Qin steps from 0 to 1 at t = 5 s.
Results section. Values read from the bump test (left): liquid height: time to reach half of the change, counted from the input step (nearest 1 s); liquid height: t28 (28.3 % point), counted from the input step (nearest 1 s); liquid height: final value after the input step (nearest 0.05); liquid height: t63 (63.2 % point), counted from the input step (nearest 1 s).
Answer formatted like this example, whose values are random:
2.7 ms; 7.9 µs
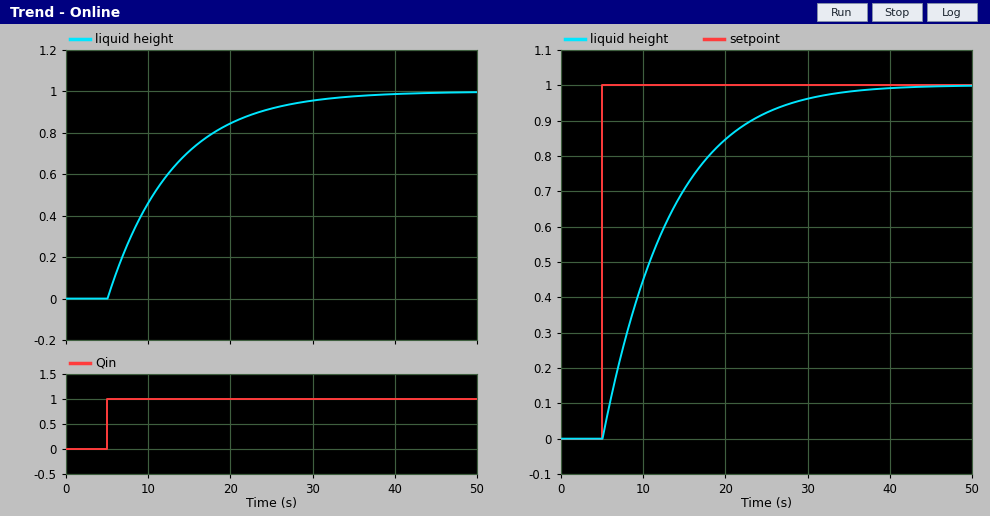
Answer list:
6 s; 3 s; 1.00; 8 s
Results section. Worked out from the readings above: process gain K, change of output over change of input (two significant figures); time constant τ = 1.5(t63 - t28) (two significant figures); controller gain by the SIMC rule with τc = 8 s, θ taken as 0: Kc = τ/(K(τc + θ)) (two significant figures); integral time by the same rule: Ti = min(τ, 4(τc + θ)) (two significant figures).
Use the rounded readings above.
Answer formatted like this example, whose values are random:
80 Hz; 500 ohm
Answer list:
1.0; 7.5 s; 0.94; 7.5 s
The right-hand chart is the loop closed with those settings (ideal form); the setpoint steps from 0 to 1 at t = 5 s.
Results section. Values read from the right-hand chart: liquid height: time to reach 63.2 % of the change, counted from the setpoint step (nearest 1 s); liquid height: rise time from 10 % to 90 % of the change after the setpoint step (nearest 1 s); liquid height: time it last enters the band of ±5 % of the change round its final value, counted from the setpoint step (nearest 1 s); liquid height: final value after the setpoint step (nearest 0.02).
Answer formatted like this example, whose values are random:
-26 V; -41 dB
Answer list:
8 s; 17 s; 23 s; 1.00
